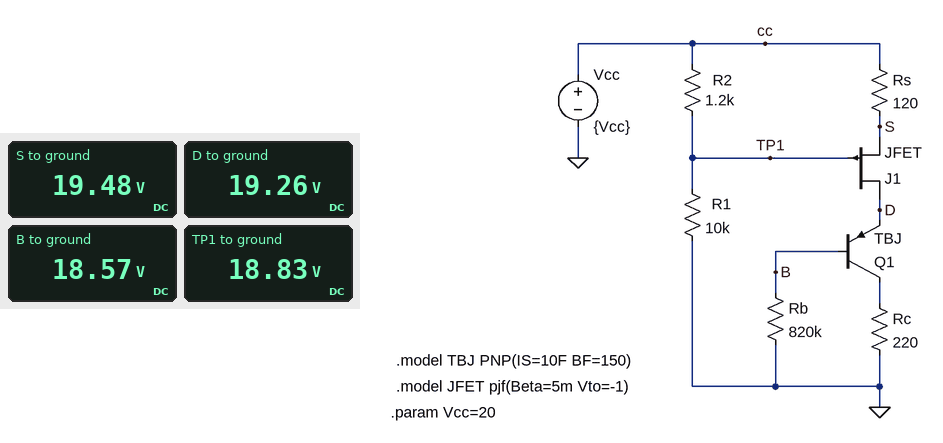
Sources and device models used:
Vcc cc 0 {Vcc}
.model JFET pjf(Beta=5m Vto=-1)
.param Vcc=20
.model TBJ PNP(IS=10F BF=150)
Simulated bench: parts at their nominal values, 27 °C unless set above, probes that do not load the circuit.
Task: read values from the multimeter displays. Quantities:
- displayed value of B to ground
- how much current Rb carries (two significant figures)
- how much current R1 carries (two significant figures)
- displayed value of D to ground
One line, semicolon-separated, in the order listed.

18.57 V; 23 µA; 1.9 mA; 19.26 V
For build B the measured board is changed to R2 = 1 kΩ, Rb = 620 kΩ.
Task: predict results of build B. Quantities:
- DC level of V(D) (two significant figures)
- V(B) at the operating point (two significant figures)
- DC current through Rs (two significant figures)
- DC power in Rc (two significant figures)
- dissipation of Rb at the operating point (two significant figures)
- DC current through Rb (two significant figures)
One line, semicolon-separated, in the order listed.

19 V; 18 V; 5.1 mA; 4.4 mW; 550 µW; 30 µA
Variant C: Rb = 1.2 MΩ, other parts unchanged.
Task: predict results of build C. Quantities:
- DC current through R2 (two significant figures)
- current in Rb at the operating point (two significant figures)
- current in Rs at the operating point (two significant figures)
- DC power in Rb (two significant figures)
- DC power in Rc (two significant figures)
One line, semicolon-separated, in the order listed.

880 µA; 16 µA; 3.4 mA; 290 µW; 1.2 mW
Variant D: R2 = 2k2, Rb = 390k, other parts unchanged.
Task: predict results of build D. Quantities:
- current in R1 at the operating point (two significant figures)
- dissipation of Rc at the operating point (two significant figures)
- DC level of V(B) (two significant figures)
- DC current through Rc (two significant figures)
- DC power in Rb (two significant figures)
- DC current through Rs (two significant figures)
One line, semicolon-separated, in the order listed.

1.8 mA; 10 mW; 18 V; 6.9 mA; 820 µW; 8.0 mA
